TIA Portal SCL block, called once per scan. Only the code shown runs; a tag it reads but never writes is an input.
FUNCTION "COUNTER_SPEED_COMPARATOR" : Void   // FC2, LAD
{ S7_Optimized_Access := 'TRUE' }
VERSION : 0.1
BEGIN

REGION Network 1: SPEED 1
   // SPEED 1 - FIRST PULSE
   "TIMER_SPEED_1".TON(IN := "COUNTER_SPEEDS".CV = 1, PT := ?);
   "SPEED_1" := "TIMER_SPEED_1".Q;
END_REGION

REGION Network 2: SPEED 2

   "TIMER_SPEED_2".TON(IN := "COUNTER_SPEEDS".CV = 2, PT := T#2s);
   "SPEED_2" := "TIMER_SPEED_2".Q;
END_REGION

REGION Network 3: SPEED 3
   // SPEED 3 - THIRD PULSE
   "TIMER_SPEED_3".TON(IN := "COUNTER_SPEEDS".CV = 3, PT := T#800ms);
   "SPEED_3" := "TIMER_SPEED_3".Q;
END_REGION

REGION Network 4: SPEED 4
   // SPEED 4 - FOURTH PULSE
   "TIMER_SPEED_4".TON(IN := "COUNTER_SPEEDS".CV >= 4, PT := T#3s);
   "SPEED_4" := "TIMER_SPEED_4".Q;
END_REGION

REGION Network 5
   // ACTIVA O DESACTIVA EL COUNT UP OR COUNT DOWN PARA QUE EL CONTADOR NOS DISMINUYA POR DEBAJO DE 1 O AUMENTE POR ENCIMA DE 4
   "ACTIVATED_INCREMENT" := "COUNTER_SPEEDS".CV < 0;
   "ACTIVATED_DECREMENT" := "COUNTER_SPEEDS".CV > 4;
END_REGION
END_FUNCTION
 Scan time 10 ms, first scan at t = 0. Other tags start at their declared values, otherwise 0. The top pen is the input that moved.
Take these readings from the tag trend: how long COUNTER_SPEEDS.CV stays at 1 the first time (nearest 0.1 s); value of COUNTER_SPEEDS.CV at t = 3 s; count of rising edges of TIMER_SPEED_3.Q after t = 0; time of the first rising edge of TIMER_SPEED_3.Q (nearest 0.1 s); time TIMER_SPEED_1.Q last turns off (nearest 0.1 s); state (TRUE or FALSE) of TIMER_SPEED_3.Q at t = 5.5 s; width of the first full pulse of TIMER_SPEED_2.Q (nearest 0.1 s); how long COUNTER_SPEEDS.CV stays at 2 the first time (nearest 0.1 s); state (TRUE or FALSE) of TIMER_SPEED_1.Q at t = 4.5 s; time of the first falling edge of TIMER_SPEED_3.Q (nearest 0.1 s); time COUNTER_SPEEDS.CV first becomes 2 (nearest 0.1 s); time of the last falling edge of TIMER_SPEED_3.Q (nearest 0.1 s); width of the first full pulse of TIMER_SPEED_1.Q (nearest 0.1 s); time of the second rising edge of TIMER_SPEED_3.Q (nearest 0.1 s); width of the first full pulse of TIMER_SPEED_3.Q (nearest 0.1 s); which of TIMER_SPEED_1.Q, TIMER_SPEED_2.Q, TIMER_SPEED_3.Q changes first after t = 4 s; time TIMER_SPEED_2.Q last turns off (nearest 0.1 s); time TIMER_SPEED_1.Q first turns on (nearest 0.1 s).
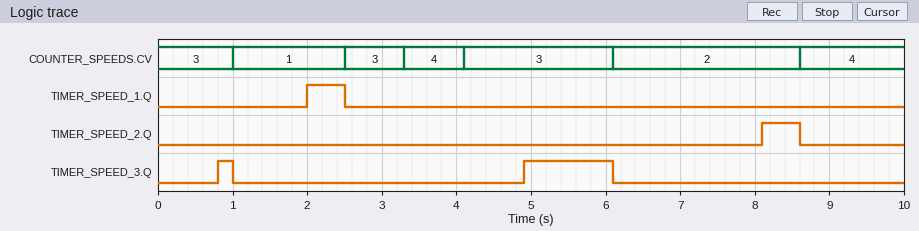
1.5 s
3
2
0.8 s
2.5 s
TRUE
0.5 s
2.5 s
FALSE
1.0 s
6.1 s
6.1 s
0.5 s
4.9 s
0.2 s
TIMER_SPEED_3.Q
8.6 s
2.0 s
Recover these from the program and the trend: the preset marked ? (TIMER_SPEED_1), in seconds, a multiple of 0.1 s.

1.0 s
